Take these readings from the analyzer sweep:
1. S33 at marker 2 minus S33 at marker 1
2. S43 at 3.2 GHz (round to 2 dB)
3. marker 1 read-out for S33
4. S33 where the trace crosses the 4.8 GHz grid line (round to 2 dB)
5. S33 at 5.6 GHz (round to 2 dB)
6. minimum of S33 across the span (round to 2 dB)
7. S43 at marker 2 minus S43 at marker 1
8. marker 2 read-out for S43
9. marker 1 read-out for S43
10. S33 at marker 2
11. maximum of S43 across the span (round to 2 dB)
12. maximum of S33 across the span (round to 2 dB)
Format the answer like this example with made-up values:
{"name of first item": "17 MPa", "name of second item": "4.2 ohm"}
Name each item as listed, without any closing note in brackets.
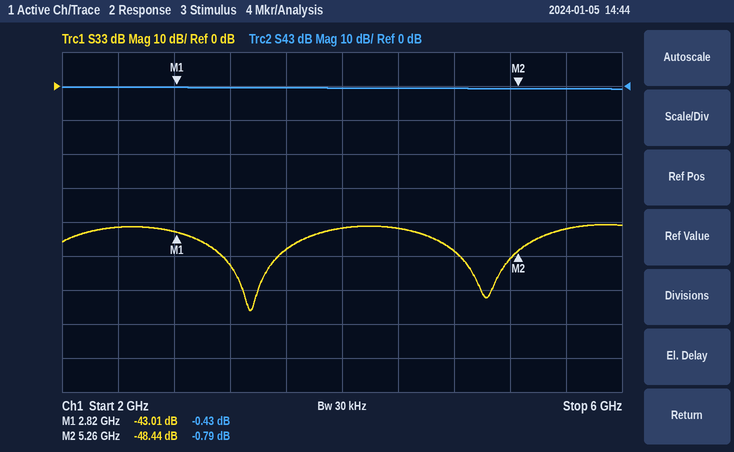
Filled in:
{"S33 at marker 2 minus S33 at marker 1": "-5.43 dB", "S43 at 3.2 GHz": "0 dB", "marker 1 read-out for S33": "-43.01 dB", "S33 where the trace crosses the 4.8 GHz grid line": "-48 dB", "S33 at 5.6 GHz": "-42 dB", "minimum of S33 across the span": "-66 dB", "S43 at marker 2 minus S43 at marker 1": "-0.36 dB", "marker 2 read-out for S43": "-0.79 dB", "marker 1 read-out for S43": "-0.43 dB", "S33 at marker 2": "-48.44 dB", "maximum of S43 across the span": "0 dB", "maximum of S33 across the span": "-40 dB"}
